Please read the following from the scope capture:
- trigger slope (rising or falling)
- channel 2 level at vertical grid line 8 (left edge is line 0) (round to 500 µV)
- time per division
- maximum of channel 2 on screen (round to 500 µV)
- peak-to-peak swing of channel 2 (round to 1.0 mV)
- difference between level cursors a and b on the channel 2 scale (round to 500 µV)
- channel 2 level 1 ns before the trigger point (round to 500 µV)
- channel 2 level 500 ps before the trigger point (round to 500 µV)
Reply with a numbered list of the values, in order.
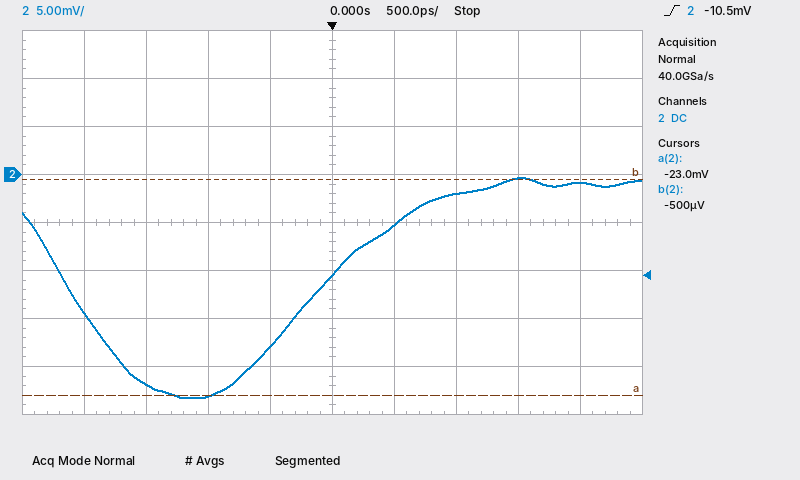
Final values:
1. rising
2. -500 µV
3. 500 ps
4. -500 µV
5. 23.0 mV
6. 22.5 mV
7. -23.0 mV
8. -18.0 mV
